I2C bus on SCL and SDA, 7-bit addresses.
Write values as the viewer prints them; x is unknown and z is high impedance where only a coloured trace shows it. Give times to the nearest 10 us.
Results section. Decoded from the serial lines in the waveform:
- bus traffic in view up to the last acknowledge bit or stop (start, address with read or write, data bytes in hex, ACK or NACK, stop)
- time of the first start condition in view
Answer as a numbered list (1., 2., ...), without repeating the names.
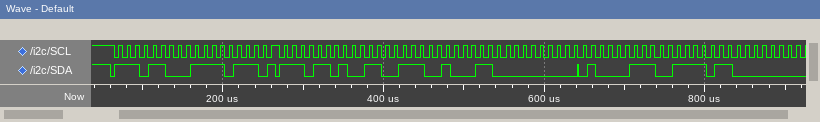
1. start, address 76 write ACK, F7 ACK, repeated start, address 76 read ACK, 67 ACK, 46 ACK, 00 ACK, 87 ACK, 7B ACK
2. 60 us
